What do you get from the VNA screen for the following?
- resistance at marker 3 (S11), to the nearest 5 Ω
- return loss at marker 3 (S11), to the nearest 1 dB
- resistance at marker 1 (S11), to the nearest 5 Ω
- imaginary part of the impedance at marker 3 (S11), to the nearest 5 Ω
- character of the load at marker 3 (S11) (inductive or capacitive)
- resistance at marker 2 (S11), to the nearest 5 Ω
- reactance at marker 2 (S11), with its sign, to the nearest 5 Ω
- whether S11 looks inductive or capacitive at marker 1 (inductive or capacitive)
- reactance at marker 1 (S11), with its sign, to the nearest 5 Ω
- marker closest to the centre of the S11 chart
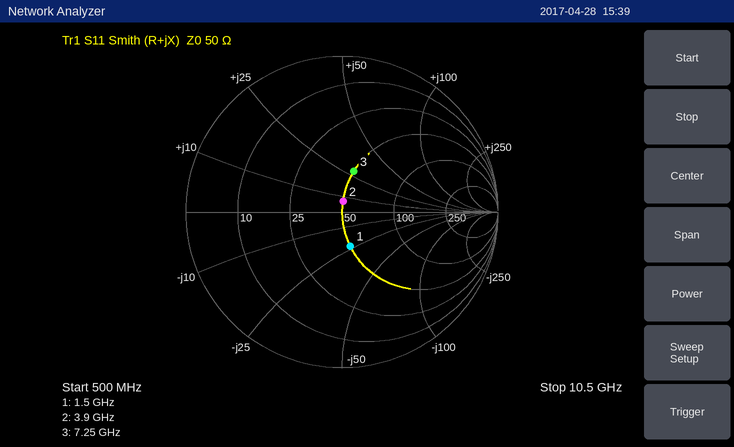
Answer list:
50 Ω
11 dB
50 Ω
+30 Ω
inductive
50 Ω
+5 Ω
capacitive
-25 Ω
marker 2
